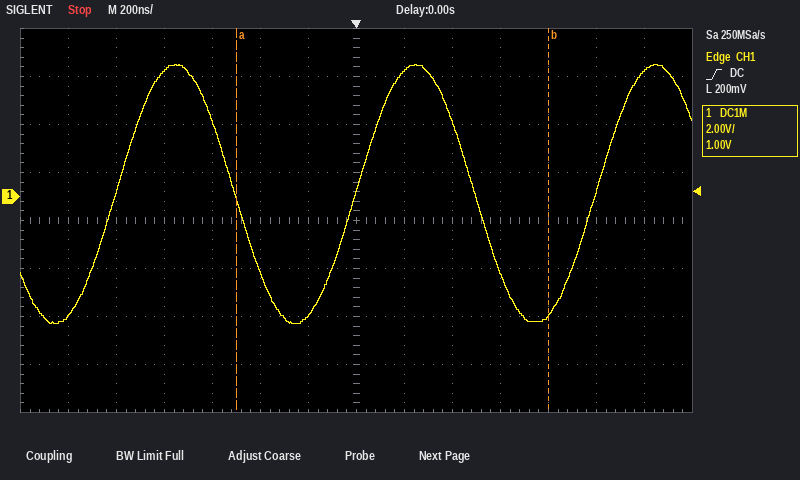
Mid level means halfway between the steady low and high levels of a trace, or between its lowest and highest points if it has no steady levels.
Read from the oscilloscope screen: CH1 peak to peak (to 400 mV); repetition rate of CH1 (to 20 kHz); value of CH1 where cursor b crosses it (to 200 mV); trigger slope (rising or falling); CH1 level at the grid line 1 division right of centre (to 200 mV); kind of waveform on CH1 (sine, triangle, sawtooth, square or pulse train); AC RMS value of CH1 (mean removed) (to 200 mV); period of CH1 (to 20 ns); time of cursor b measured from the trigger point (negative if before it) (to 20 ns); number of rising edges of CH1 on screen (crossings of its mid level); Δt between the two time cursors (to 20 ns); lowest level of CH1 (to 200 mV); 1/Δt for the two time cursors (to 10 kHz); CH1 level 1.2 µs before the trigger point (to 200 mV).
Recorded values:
10.8 V
1.00 MHz
-5.0 V
rising
5.2 V
sine
3.8 V
1.00 µs
+800 ns
3
1.30 µs
-5.2 V
770 kHz
-5.0 V
